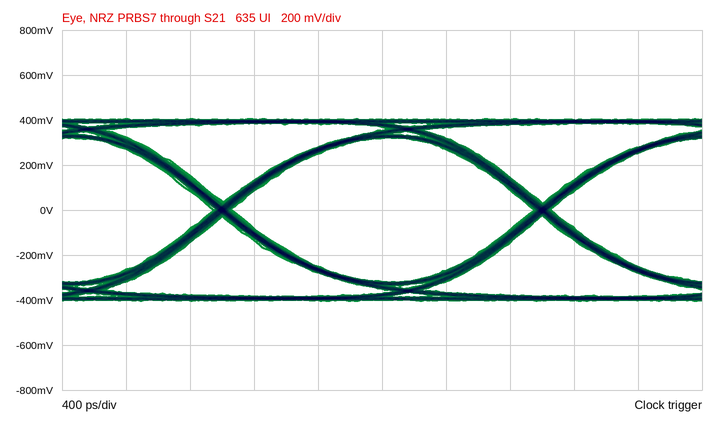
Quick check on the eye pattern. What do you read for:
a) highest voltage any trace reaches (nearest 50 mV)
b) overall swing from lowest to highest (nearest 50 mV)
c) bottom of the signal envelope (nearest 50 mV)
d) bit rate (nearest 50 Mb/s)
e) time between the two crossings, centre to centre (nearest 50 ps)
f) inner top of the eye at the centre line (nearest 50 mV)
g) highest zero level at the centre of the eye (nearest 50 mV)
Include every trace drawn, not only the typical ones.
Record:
400 mV
800 mV
-400 mV
500 Mb/s
2.00 ns
300 mV
-300 mV
